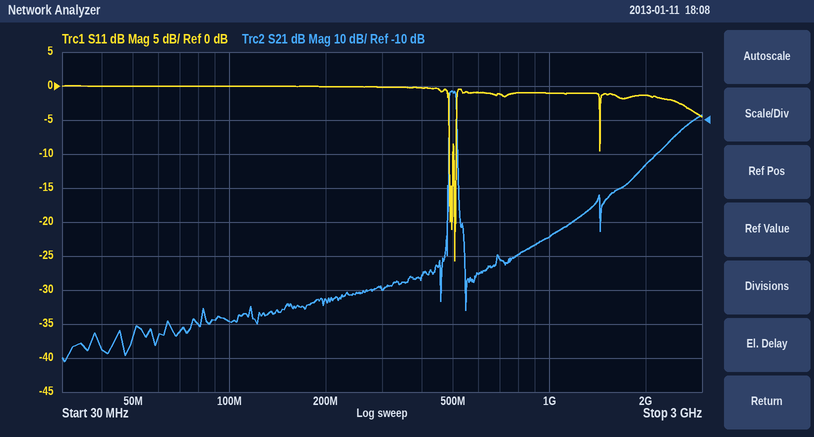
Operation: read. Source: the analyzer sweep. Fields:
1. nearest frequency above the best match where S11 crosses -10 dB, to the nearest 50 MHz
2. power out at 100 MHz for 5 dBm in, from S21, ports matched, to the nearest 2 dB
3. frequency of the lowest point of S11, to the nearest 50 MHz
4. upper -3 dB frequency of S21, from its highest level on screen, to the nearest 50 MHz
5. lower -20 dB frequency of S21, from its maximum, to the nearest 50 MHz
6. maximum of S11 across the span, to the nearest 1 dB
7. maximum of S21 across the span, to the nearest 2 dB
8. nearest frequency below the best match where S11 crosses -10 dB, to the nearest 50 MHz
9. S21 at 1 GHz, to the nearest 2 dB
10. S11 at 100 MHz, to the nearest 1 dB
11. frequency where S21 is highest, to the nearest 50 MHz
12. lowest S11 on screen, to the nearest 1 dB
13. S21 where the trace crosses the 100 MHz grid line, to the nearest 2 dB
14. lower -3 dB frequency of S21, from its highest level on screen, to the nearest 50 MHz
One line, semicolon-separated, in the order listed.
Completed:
500 MHz; -64 dBm; 500 MHz; 500 MHz; 500 MHz; 0 dB; -2 dB; 500 MHz; -44 dB; 0 dB; 500 MHz; -26 dB; -70 dB; 500 MHz
